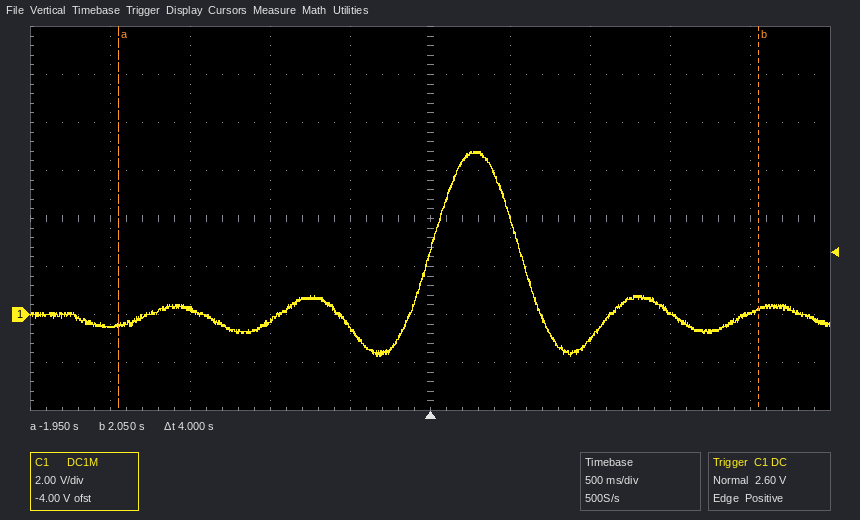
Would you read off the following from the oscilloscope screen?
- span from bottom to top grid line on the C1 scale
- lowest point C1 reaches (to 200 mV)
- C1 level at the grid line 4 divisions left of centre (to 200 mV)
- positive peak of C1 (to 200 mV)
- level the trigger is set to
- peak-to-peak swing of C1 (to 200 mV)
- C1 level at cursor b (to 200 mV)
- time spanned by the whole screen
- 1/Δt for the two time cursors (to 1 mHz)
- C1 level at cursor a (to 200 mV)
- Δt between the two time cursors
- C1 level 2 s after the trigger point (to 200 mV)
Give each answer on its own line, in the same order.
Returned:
16 V
-1.8 V
-600 mV
6.8 V
2.60 V
8.6 V
200 mV
5 s
250 mHz
-400 mV
4 s
0.0 V
